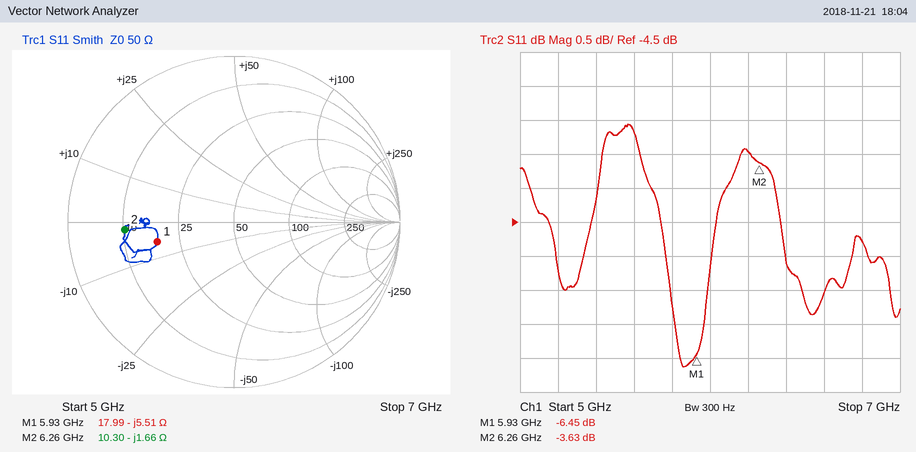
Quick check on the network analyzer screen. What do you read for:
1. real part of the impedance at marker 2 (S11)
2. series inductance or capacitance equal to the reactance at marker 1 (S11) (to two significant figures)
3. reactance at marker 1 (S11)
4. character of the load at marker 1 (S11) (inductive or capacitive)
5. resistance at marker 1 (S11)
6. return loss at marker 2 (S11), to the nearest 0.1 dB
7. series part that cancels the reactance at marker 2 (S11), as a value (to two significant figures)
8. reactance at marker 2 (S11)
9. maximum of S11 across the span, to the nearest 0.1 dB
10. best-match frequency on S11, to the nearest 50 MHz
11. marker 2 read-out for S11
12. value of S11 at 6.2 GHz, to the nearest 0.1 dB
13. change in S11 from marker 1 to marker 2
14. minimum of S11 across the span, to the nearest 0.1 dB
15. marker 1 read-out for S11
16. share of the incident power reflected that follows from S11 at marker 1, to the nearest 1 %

10.30 Ω
4.9 pF
-5.51 Ω
capacitive
17.99 Ω
3.6 dB
42 pH
-1.66 Ω
-3.1 dB
5.85 GHz
-3.63 dB
-3.5 dB
2.82 dB
-6.6 dB
-6.45 dB
23 %
